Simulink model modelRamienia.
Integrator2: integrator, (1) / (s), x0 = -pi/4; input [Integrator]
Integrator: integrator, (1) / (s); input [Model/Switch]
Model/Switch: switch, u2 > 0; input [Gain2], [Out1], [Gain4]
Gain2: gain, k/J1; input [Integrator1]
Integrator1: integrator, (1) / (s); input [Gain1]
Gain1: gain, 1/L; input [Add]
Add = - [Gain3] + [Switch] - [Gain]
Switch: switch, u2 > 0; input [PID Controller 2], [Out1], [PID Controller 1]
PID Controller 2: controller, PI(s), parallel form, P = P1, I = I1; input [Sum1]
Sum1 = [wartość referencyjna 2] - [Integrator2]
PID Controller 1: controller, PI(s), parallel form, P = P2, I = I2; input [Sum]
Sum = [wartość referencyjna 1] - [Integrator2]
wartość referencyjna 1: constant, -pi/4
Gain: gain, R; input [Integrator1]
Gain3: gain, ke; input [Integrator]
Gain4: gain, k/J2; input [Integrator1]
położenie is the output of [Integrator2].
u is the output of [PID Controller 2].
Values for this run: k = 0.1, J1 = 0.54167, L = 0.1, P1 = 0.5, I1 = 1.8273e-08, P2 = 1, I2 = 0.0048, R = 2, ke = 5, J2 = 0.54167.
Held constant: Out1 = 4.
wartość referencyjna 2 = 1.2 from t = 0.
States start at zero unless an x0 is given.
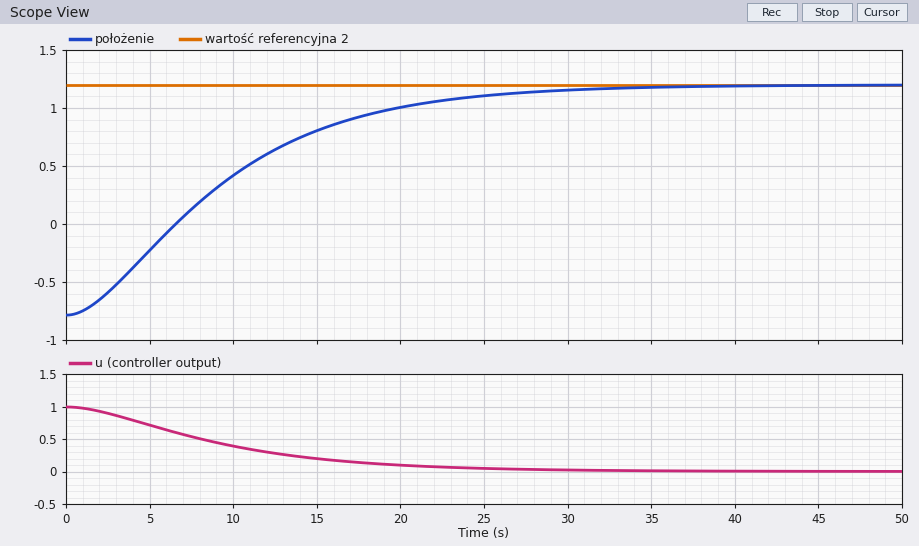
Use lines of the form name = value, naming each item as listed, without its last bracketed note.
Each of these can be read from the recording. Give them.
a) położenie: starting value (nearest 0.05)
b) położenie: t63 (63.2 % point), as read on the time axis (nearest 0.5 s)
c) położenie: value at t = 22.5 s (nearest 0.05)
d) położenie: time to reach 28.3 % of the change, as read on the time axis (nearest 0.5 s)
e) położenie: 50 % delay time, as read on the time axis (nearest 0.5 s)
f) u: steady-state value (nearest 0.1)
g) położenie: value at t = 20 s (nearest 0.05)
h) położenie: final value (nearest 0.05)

położenie: starting value = -0.80
położenie: t63 (63.2 % point), as read on the time axis = 10.5 s
położenie: value at t = 22.5 s = 1.05
położenie: time to reach 28.3 % of the change, as read on the time axis = 5.0 s
położenie: 50 % delay time, as read on the time axis = 8.0 s
u: steady-state value = 0.0
położenie: value at t = 20 s = 1.00
położenie: final value = 1.20
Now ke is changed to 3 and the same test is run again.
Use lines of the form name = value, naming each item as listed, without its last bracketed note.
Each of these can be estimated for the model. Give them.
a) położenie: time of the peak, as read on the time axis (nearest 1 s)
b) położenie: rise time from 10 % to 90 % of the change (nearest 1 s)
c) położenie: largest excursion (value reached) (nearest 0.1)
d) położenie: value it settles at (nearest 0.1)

położenie: time of the peak, as read on the time axis = 19 s
położenie: rise time from 10 % to 90 % of the change = 9 s
położenie: largest excursion (value reached) = 1.3
położenie: value it settles at = 1.2
